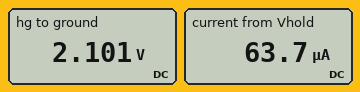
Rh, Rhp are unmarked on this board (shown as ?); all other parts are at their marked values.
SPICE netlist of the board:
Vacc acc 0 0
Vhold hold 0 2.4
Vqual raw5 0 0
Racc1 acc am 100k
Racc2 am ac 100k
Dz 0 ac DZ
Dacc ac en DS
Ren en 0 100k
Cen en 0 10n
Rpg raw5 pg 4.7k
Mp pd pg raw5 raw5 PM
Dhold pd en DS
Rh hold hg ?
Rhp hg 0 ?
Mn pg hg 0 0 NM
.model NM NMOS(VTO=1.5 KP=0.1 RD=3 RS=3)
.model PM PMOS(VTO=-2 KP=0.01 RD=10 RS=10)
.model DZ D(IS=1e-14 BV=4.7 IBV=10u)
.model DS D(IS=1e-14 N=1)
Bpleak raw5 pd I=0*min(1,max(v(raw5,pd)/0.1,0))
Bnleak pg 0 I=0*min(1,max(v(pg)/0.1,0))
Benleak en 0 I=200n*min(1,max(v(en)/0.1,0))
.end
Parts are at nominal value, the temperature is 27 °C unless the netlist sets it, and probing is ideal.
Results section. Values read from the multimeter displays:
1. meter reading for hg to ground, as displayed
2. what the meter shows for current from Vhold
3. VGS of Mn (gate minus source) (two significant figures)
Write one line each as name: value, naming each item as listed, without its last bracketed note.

meter reading for hg to ground, as displayed: 2.101 V
what the meter shows for current from Vhold: 63.7 µA
VGS of Mn (gate minus source): 2.1 V
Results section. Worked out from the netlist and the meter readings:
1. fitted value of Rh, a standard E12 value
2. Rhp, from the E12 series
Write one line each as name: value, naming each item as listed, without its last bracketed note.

fitted value of Rh, a standard E12 value: 4.7 kΩ
Rhp, from the E12 series: 33 kΩ
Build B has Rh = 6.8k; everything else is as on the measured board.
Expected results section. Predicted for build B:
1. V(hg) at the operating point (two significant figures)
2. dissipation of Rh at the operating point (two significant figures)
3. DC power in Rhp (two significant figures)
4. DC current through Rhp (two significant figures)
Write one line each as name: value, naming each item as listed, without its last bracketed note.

V(hg) at the operating point: 2.0 V
dissipation of Rh at the operating point: 25 µW
DC power in Rhp: 120 µW
DC current through Rhp: 60 µA
